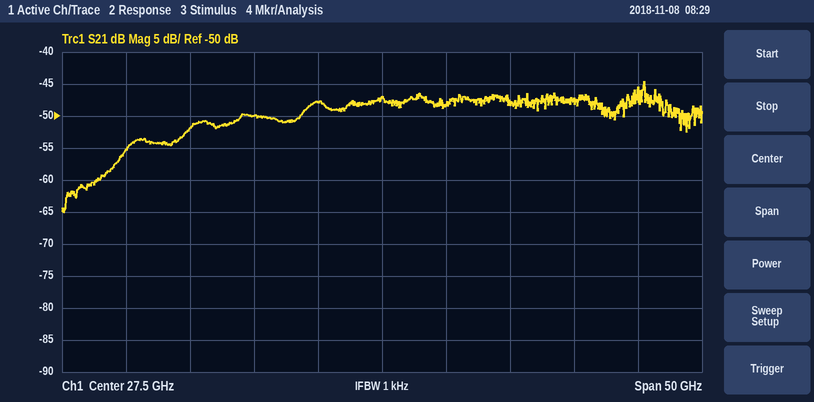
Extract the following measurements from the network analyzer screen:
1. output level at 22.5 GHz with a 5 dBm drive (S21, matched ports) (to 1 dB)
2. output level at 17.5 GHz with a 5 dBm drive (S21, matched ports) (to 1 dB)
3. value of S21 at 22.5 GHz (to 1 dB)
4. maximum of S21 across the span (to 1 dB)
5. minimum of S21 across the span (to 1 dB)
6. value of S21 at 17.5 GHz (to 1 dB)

-43 dBm
-45 dBm
-48 dB
-45 dB
-65 dB
-50 dB
